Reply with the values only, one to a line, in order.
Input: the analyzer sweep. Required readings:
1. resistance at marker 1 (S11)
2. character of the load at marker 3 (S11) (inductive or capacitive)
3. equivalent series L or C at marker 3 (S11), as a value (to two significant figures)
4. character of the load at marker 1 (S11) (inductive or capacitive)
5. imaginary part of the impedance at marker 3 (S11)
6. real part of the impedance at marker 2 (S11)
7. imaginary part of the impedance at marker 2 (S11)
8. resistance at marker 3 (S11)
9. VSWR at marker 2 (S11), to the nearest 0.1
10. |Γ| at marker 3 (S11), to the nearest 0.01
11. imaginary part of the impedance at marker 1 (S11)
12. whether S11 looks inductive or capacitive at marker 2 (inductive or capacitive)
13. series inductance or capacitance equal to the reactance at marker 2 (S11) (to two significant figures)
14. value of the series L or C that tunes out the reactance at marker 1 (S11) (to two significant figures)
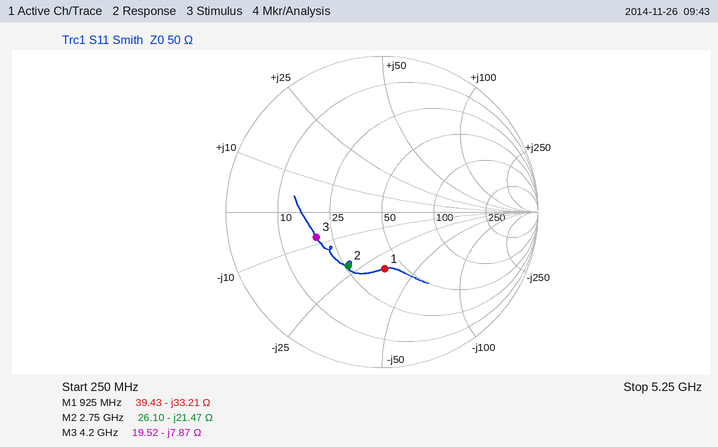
39.43 Ω
capacitive
4.8 pF
capacitive
-7.87 Ω
26.10 Ω
-21.47 Ω
19.52 Ω
2.4
0.45
-33.21 Ω
capacitive
2.7 pF
5.7 nH
